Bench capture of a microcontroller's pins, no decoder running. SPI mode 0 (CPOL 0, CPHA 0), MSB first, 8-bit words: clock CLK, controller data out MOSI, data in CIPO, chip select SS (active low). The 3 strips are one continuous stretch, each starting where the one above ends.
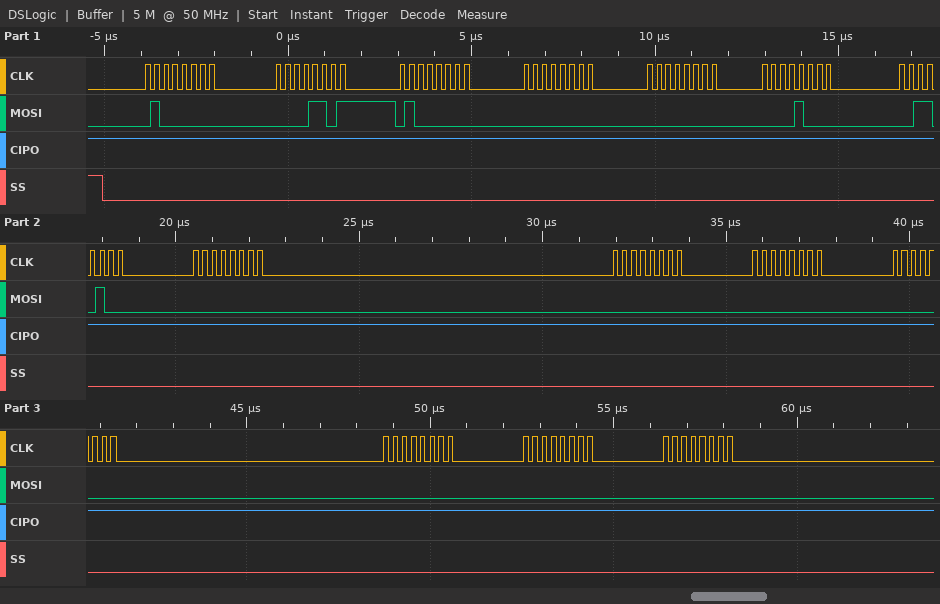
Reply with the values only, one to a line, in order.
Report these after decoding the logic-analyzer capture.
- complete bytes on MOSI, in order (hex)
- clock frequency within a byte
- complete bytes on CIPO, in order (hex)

40 0D 40 00 00 08 34 00 00 00 00 00 00 00
4 MHz
FF FF FF FF FF FF FF FF FF FF FF FF FF FF
